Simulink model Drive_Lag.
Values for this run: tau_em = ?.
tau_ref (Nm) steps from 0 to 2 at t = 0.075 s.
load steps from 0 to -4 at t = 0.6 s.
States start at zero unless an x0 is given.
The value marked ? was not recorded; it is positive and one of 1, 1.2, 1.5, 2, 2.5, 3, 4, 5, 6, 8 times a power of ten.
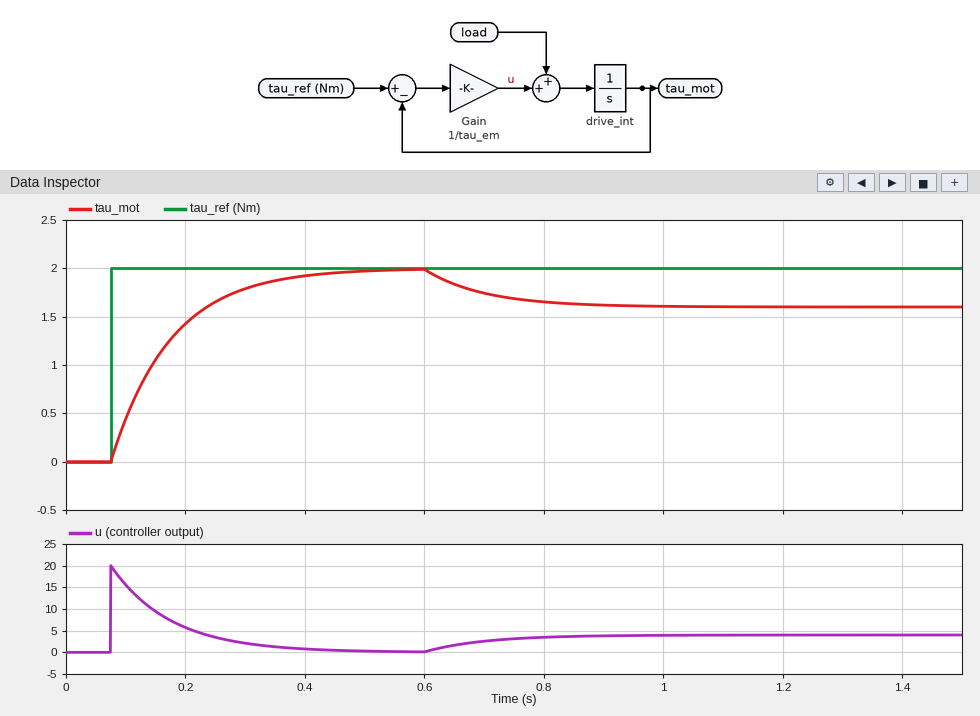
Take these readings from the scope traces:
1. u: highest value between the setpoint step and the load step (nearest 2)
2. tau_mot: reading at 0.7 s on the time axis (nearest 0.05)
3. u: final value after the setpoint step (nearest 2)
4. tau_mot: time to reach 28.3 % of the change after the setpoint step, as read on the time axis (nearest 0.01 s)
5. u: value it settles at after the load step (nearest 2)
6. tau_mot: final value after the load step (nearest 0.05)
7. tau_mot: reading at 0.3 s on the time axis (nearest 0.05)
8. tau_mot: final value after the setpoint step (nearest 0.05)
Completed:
20
1.75
0
0.11 s
4
1.60
1.80
2.00
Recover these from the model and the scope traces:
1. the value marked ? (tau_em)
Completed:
0.1
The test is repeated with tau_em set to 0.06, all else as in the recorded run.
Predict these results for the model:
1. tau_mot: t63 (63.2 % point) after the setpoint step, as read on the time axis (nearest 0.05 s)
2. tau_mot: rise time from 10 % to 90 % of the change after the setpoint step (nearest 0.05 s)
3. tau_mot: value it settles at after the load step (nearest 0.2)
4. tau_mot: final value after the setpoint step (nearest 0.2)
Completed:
0.15 s
0.15 s
1.8
2.0
